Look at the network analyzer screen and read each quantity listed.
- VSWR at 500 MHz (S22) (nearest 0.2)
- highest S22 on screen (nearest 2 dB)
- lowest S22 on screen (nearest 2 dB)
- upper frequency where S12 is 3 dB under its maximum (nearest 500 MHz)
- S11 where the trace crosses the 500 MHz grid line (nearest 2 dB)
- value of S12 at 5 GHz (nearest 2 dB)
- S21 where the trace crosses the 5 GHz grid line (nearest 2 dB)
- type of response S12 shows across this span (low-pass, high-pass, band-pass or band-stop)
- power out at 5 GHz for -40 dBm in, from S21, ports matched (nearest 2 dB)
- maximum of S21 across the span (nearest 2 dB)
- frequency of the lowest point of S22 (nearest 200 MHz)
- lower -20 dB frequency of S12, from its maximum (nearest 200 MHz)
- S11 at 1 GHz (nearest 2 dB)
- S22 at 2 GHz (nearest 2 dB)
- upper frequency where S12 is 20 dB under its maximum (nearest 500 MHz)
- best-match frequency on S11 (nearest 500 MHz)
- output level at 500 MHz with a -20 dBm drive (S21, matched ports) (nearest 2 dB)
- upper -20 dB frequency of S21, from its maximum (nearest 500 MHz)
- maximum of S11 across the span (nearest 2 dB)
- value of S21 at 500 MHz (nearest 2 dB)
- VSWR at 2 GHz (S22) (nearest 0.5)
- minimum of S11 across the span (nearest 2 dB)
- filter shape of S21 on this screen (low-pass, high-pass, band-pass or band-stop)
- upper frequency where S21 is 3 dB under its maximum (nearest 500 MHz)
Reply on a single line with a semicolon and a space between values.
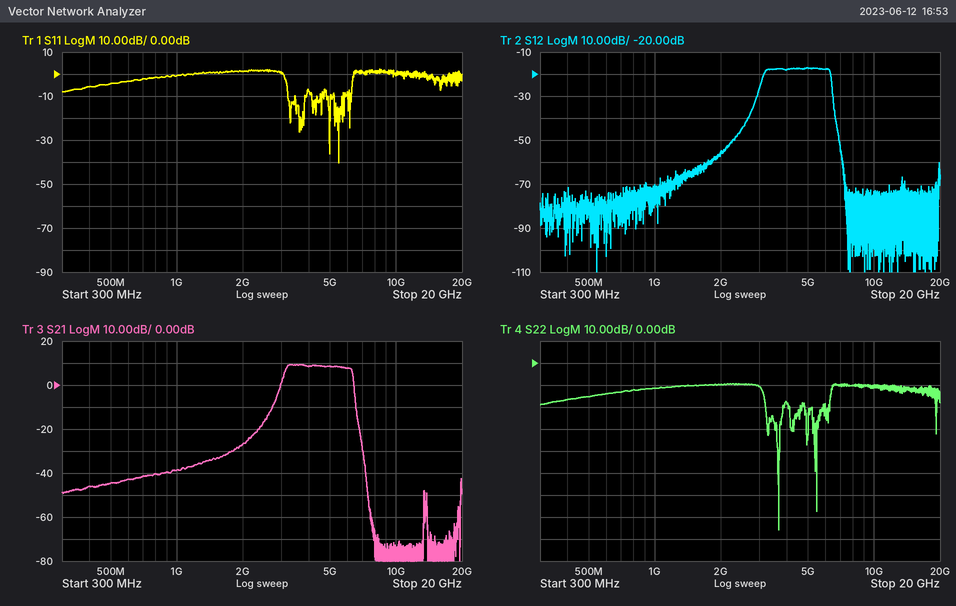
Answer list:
1.4; -10 dB; -76 dB; 6.5 GHz; -4 dB; -18 dB; 8 dB; band-pass; -32 dBm; 10 dB; 3.6 GHz; 2.8 GHz; 0 dB; -10 dB; 6.5 GHz; 5.5 GHz; -64 dBm; 6.5 GHz; 2 dB; -44 dB; 2.0; -40 dB; band-pass; 6.5 GHz
